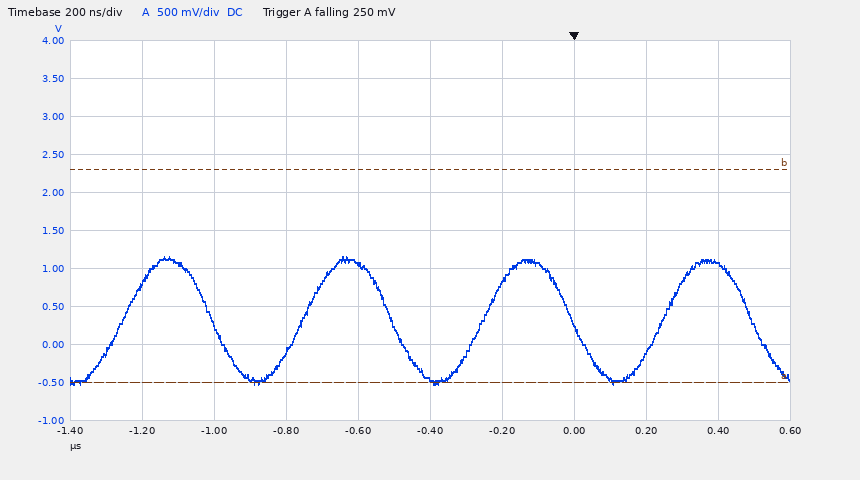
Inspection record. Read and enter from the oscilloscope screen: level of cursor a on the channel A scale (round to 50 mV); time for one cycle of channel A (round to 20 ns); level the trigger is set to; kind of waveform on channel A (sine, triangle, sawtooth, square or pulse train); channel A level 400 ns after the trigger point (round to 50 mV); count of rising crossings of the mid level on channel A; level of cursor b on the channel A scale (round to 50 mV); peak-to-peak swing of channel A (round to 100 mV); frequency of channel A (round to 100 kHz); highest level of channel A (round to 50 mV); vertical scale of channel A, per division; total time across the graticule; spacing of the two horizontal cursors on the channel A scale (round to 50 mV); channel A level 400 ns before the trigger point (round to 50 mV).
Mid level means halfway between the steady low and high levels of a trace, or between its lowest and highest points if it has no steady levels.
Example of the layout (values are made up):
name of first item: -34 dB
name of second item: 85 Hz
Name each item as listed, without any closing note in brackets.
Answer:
level of cursor a on the channel A scale: -500 mV
time for one cycle of channel A: 500 ns
level the trigger is set to: 250 mV
kind of waveform on channel A: sine
channel A level 400 ns after the trigger point: 1.05 V
count of rising crossings of the mid level on channel A: 4
level of cursor b on the channel A scale: 2.30 V
peak-to-peak swing of channel A: 1.70 V
frequency of channel A: 2.0 MHz
highest level of channel A: 1.15 V
vertical scale of channel A, per division: 500 mV
total time across the graticule: 2 µs
spacing of the two horizontal cursors on the channel A scale: 2.80 V
channel A level 400 ns before the trigger point: -450 mV
